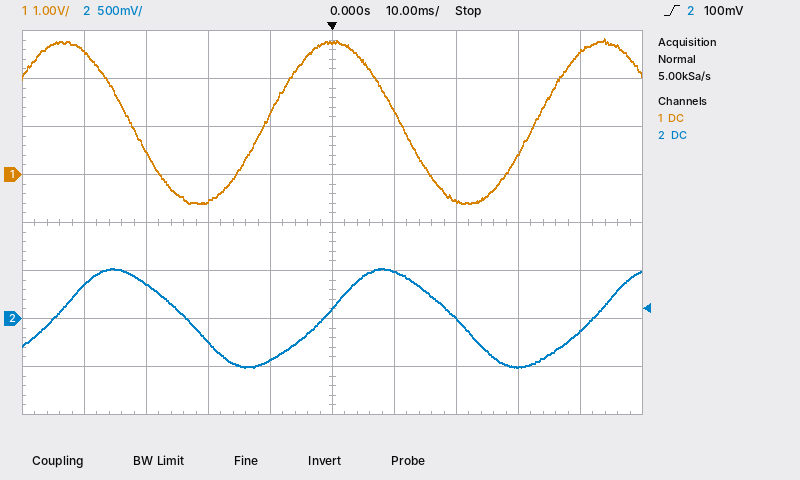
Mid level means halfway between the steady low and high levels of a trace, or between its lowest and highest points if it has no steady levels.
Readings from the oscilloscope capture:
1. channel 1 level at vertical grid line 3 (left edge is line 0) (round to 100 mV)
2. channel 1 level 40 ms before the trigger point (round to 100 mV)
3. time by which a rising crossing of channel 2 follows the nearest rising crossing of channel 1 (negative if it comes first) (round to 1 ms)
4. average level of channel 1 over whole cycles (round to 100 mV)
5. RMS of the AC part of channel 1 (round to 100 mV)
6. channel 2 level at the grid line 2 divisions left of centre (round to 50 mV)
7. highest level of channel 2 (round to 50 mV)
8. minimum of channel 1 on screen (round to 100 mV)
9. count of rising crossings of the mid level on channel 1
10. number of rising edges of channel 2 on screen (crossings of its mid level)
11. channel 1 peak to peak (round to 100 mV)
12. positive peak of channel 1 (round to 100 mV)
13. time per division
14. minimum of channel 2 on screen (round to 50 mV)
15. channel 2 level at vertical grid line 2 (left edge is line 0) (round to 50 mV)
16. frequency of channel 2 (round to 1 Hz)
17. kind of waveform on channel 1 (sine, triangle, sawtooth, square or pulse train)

-600 mV
2.6 V
+9 ms
1.1 V
1.2 V
-250 mV
500 mV
-600 mV
2
3
3.4 V
2.8 V
10 ms
-500 mV
350 mV
23 Hz
sine
